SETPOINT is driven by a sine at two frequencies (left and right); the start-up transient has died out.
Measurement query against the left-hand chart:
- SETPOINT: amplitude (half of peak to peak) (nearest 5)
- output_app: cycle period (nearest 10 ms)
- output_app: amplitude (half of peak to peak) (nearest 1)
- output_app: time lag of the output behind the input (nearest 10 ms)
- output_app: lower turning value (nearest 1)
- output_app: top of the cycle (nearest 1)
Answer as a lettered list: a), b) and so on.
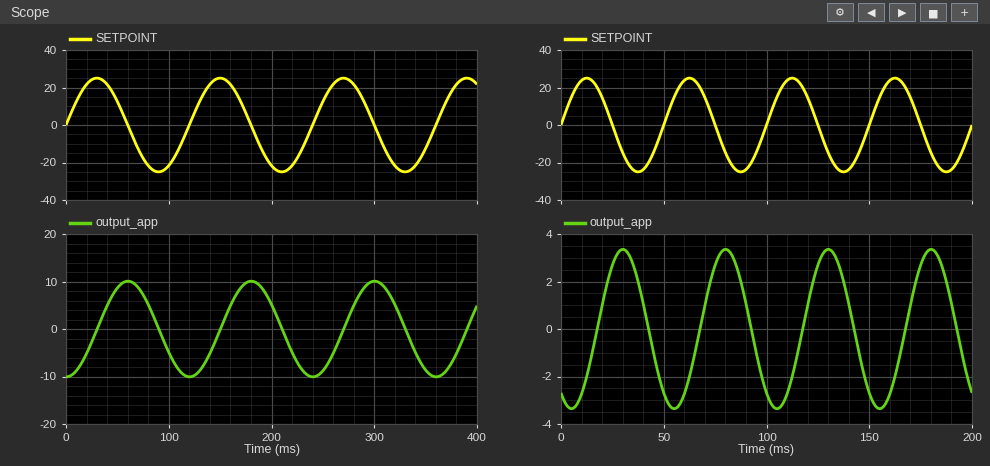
a) 25
b) 120 ms
c) 10
d) 30 ms
e) -10
f) 10
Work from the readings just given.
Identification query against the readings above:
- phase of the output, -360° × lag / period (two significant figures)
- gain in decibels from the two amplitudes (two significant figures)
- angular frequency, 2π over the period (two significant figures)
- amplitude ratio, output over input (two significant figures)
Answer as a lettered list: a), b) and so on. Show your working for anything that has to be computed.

a) -360 × 30 / 120 = -90°
b) 20 log10(10 / 25) = -8.0 dB
c) 2π / 120 = 0.052 rad/ms
d) 10 / 25 = 0.40
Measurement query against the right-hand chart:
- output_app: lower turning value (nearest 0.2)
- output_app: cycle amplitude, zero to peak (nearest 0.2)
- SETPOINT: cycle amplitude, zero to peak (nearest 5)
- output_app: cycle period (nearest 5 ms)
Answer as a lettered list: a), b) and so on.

a) -3.4
b) 3.4
c) 25
d) 50 ms
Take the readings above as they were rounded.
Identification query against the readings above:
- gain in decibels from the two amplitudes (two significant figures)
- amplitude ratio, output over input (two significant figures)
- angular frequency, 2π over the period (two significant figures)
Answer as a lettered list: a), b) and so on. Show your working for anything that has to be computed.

a) 20 log10(3.4 / 25) = -17 dB
b) 3.4 / 25 = 0.14
c) 2π / 50 = 0.13 rad/ms
